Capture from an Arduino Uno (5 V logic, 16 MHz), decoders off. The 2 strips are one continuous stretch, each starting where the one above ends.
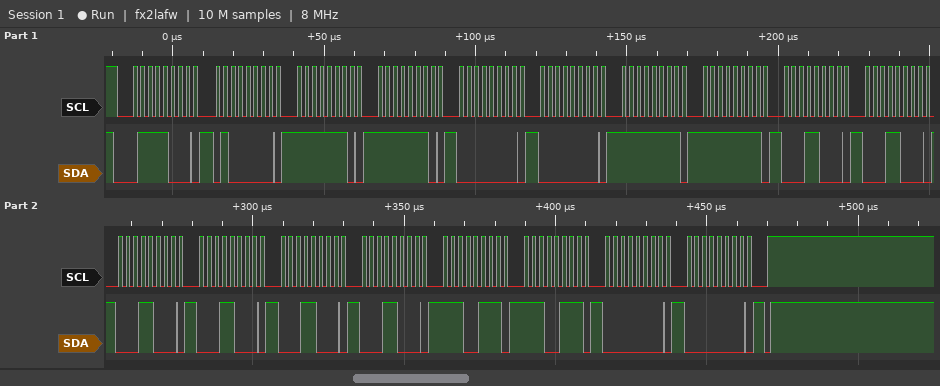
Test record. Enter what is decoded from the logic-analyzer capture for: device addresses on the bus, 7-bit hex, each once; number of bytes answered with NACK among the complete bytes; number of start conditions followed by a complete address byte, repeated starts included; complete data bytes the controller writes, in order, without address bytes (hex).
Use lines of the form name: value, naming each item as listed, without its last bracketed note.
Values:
device addresses on the bus, 7-bit hex, each once: 0x3C
number of bytes answered with NACK among the complete bytes: 0
number of start conditions followed by a complete address byte, repeated starts included: 1
complete data bytes the controller writes, in order, without address bytes: 40 FE FE 00 00 FF FF 18 18 18 18 18 18 E7 E7 00 00
